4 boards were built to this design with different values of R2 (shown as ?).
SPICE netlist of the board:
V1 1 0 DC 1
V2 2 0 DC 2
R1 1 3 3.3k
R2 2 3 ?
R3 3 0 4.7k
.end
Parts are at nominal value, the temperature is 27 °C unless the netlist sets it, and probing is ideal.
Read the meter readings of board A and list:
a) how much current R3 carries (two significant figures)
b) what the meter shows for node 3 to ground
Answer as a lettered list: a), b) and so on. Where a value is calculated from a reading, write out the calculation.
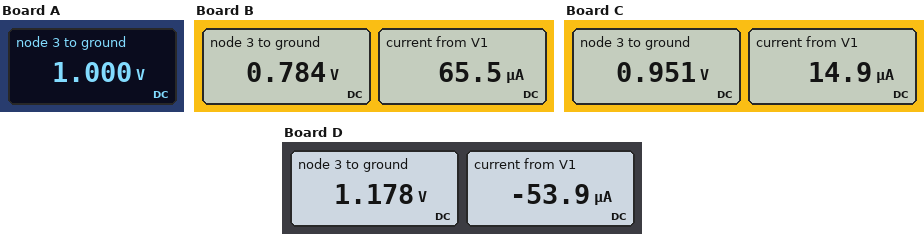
a) (1 V) / 4.7 kΩ = 210 µA
b) 1.000 V
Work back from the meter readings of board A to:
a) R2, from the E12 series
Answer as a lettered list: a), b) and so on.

a) 4.7 kΩ
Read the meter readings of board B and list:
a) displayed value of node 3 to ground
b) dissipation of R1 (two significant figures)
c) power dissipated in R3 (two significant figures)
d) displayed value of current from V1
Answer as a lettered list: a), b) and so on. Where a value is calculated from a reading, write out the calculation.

a) 0.784 V
b) (1 V - 784 mV)^2 / 3.3 kΩ = 14 µW
c) (784 mV)^2 / 4.7 kΩ = 130 µW
d) 65.5 µA
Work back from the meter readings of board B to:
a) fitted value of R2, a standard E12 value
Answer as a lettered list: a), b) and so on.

a) 12 kΩ
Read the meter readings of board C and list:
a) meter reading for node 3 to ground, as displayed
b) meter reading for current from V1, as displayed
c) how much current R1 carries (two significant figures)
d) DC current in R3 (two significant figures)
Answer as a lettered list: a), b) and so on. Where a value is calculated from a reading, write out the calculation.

a) 0.951 V
b) 14.9 µA
c) (1 V - 951 mV) / 3.3 kΩ = 15 µA
d) (951 mV) / 4.7 kΩ = 200 µA
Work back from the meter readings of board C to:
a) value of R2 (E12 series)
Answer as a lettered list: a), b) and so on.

a) 5.6 kΩ
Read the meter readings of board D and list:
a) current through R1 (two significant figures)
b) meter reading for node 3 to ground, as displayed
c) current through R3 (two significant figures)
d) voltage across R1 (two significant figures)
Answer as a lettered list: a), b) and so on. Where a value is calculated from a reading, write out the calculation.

a) (1.178 V - 1 V) / 3.3 kΩ = 54 µA
b) 1.178 V
c) (1.178 V) / 4.7 kΩ = 250 µA
d) 1.178 V - 1 V = 180 mV
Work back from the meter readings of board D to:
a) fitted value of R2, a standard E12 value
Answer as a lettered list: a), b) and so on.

a) 2.7 kΩ
